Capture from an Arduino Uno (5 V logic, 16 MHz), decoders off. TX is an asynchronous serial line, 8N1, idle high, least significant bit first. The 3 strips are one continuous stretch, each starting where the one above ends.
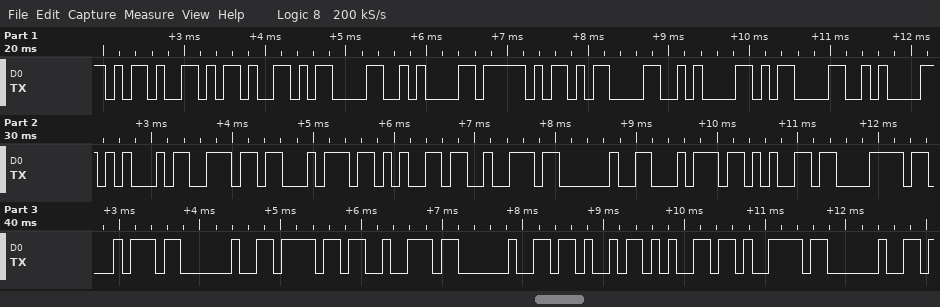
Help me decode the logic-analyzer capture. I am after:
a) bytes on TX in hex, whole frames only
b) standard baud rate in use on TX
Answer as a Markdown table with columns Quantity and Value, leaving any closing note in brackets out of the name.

| Quantity | Value |
|---|---|
| bytes on TX in hex, whole frames only | 0x2D 0x2D 0x0D 0x0A 0x5F 0x0D 0x0A 0x0D 0x0A 0x45 0x6E 0x74 0x65 0x72 0x20 0x74 0x65 0x78 0x74 0x20 0x6F 0x72 0x20 0x4B 0x65 0x79 0x20 |
| standard baud rate in use on TX | 9600 baud |
